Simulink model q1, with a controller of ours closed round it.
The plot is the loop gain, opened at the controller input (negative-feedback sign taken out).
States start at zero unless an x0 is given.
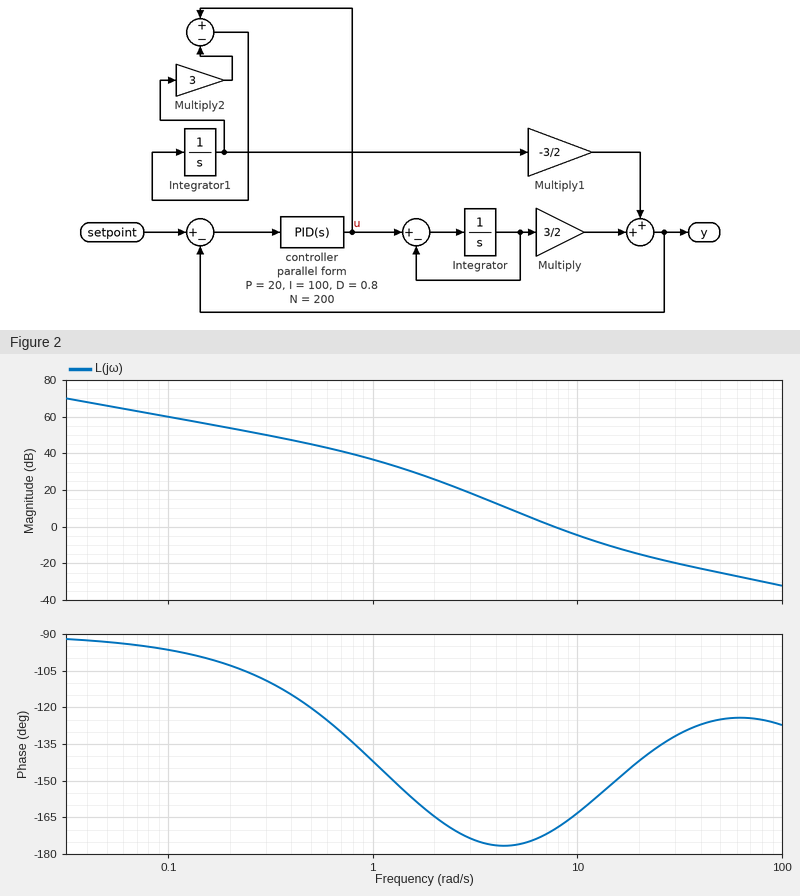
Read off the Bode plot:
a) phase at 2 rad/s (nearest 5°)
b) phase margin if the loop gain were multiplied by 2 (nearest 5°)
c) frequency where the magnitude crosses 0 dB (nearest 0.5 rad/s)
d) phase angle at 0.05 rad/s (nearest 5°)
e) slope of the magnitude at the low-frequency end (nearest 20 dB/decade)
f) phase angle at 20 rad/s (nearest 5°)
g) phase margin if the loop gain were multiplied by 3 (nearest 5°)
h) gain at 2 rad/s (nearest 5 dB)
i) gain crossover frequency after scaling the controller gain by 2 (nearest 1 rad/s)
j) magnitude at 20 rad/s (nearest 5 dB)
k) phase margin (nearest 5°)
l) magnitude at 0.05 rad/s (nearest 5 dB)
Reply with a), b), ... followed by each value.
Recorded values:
a) -165°
b) 20°
c) 7.5 rad/s
d) -95°
e) -20 dB/decade
f) -140°
g) 25°
h) 25 dB
i) 11 rad/s
j) -15 dB
k) 10°
l) 65 dB
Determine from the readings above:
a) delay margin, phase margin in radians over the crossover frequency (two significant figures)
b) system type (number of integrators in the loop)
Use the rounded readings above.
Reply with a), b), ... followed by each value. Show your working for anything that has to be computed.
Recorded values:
a) 10 × π / 180 / 7.5 = 0.023 s
b) 1
